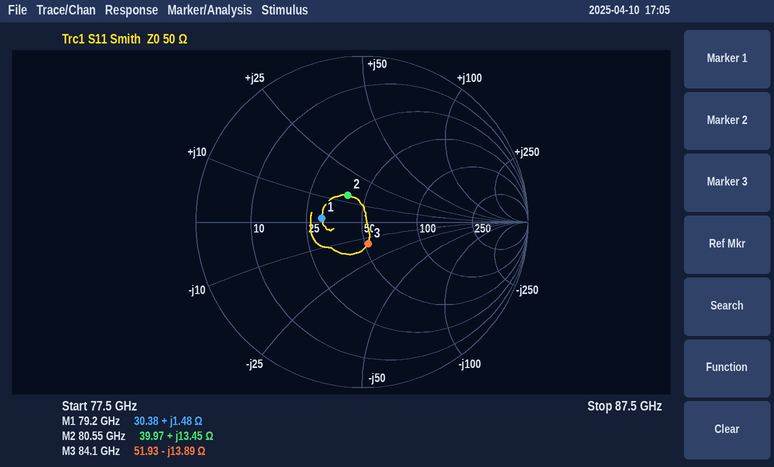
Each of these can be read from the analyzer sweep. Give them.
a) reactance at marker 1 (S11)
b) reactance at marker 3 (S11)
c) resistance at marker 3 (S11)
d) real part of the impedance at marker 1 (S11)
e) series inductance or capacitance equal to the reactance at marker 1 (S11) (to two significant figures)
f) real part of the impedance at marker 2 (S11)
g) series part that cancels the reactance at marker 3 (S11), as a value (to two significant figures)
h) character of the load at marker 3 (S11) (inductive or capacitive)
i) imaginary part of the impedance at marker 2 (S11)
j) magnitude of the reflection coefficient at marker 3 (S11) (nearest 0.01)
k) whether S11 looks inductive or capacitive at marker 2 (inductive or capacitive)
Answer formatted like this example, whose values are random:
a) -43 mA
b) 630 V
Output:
a) +1.48 Ω
b) -13.89 Ω
c) 51.93 Ω
d) 30.38 Ω
e) 3.0 pH
f) 39.97 Ω
g) 26 pH
h) capacitive
i) +13.45 Ω
j) 0.14
k) inductive
